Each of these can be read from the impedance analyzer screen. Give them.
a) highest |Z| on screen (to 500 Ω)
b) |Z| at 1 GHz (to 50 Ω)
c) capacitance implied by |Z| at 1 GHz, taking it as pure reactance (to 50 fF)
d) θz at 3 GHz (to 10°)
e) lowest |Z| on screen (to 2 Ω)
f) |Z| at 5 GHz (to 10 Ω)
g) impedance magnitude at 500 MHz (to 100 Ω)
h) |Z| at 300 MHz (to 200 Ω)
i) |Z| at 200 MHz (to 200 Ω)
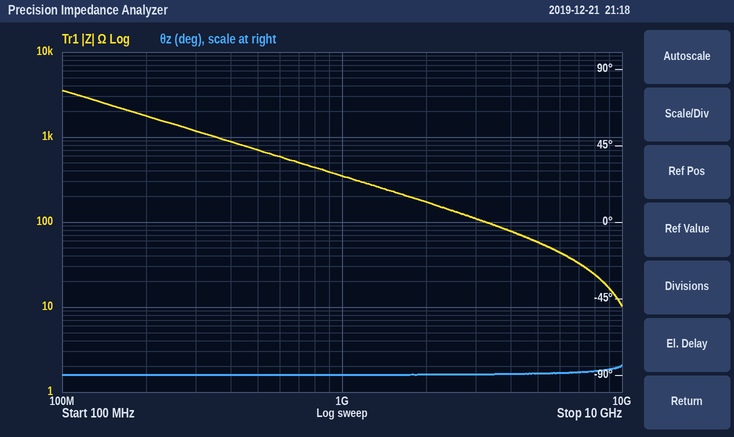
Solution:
3.5 kΩ
350 Ω
450 fF
-90°
10 Ω
60 Ω
700 Ω
1.2 kΩ
1.8 kΩ
